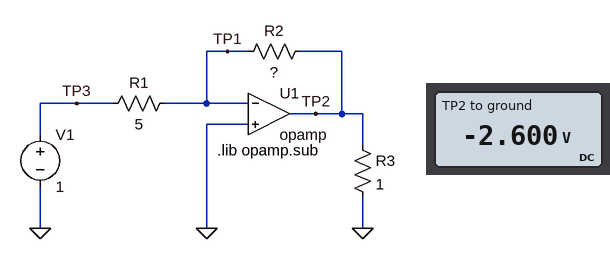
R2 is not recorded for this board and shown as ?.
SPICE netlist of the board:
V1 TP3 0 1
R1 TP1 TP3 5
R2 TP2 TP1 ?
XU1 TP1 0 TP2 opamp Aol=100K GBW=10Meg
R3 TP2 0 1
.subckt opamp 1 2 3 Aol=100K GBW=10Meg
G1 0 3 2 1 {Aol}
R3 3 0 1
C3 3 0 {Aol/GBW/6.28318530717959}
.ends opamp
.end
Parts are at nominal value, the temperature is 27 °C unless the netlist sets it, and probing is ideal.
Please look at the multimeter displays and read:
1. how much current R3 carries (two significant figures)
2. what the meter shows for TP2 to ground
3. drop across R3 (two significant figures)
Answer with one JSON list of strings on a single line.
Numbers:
["2.6 A", "-2.600 V", "2.6 V"]
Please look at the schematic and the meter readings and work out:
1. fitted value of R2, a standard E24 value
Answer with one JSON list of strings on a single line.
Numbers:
["13 Ω"]
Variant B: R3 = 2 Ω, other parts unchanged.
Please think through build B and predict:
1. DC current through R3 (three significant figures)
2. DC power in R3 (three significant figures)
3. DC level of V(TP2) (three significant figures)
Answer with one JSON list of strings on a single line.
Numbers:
["1.30 A", "3.38 W", "-2.60 V"]
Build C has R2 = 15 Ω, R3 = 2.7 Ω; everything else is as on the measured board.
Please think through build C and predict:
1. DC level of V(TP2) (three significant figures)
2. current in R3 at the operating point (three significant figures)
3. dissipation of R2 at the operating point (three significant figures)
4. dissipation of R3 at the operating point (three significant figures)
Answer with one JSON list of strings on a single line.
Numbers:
["-3.00 V", "1.11 A", "600 mW", "3.33 W"]
